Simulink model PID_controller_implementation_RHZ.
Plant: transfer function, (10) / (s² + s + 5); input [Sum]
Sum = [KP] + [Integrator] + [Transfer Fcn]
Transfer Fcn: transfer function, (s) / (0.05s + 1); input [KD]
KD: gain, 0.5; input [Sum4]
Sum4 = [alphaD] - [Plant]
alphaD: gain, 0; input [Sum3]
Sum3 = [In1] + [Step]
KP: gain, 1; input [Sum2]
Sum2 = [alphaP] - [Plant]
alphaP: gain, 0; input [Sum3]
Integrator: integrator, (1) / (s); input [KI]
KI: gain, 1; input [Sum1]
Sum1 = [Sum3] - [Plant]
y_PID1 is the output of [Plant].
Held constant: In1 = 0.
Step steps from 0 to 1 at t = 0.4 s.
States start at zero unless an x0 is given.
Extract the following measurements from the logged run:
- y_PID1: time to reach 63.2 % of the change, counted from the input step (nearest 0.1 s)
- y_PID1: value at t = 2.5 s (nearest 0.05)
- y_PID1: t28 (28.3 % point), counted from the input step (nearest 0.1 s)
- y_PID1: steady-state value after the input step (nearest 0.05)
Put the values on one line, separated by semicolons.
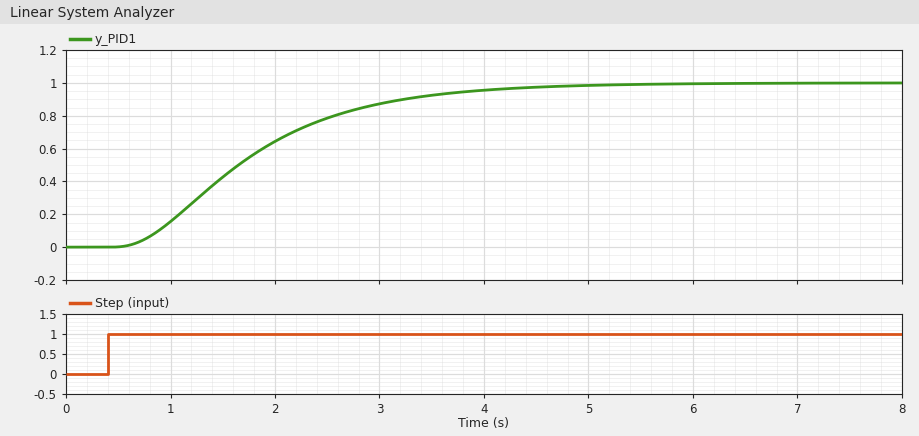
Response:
1.6 s; 0.80; 0.8 s; 1.00
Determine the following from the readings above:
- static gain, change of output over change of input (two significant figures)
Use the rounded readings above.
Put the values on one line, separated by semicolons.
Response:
1.0
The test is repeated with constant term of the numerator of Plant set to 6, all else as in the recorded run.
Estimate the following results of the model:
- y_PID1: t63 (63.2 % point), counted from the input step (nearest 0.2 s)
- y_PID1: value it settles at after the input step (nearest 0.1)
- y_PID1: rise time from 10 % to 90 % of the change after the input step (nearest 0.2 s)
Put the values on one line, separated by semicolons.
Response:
1.8 s; 1.0; 3.2 s
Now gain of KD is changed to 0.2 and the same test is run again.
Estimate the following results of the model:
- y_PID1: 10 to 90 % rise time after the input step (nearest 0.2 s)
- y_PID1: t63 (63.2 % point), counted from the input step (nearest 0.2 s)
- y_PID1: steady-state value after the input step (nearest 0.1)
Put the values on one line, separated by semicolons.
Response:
2.6 s; 1.4 s; 1.0
